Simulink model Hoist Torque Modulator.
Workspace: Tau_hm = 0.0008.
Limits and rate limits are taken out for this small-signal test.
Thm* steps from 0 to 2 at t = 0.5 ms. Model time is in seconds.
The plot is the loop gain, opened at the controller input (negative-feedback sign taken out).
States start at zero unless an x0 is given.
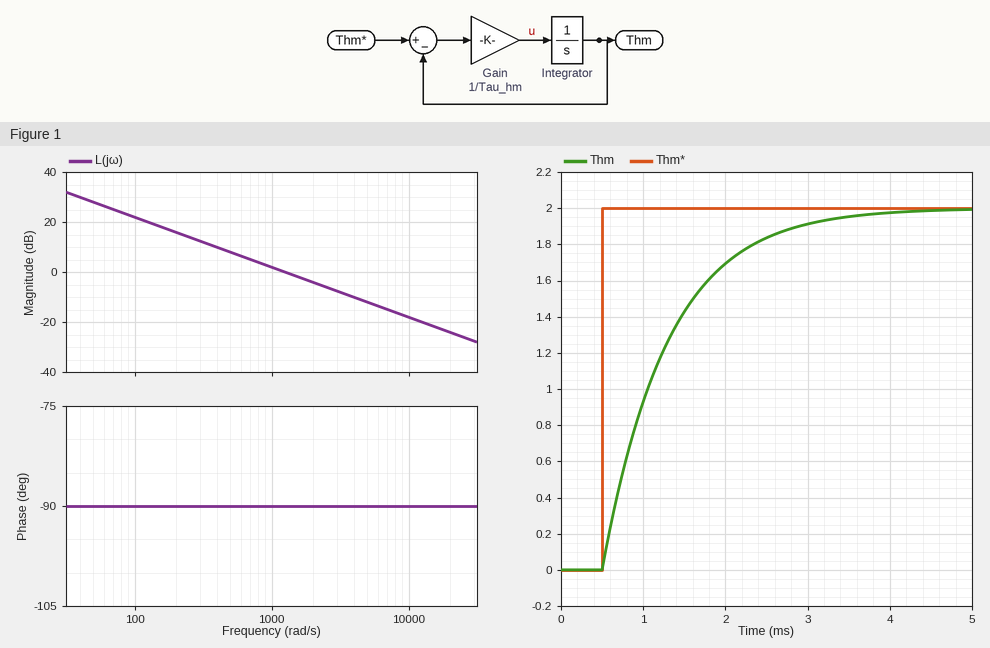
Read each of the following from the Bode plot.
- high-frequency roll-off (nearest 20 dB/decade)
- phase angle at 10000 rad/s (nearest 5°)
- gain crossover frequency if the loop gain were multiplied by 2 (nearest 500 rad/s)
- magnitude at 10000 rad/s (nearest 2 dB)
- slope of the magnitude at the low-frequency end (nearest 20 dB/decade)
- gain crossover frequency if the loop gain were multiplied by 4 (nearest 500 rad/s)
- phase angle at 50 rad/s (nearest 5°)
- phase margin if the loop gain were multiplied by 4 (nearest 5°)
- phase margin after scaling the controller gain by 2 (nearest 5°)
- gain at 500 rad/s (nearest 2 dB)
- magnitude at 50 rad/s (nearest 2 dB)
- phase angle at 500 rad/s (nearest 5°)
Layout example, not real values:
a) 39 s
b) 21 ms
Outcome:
a) -20 dB/decade
b) -90°
c) 2500 rad/s
d) -18 dB
e) -20 dB/decade
f) 5000 rad/s
g) -90°
h) 90°
i) 90°
j) 8 dB
k) 28 dB
l) -90°
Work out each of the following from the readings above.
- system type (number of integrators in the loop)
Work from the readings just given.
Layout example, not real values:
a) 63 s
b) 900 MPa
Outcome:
a) 1
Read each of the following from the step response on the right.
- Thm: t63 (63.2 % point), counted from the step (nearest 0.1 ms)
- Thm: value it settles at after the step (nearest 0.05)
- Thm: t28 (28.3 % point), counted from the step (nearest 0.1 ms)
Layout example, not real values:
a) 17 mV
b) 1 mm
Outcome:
a) 0.8 ms
b) 2.00
c) 0.3 ms
